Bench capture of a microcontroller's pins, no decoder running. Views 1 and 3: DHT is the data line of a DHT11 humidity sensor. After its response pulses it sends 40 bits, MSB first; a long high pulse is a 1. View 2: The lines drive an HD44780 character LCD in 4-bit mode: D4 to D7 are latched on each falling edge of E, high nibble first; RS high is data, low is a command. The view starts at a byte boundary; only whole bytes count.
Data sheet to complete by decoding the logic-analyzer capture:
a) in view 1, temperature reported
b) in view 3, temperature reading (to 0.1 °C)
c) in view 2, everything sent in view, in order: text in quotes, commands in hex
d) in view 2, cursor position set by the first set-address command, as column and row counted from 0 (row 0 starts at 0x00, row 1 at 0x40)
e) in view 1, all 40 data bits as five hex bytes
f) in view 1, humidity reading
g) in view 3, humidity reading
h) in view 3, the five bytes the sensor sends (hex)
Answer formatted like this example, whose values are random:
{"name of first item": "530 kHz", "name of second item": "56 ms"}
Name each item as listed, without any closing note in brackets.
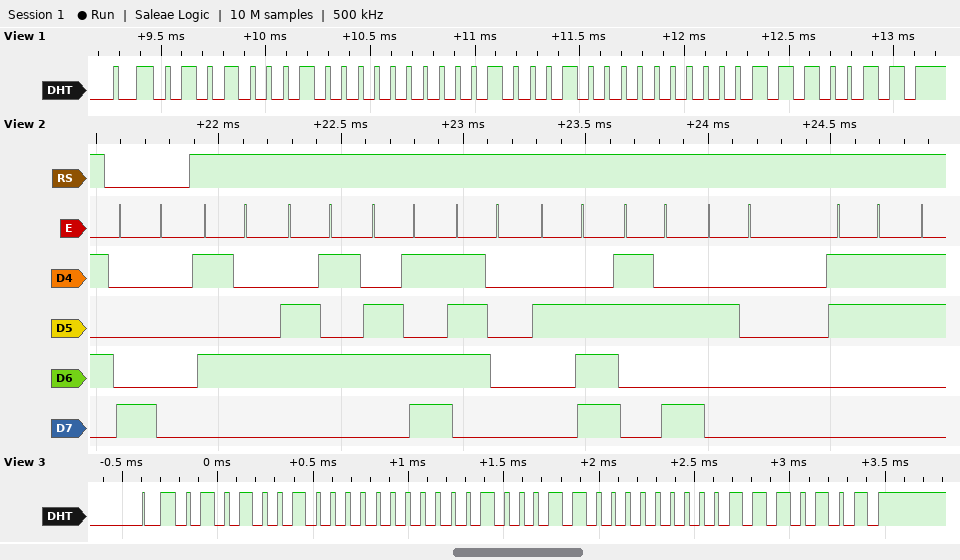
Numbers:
{"in view 1, temperature reported": "34.0 °C", "in view 3, temperature reading": "35.0 °C", "in view 2, everything sent in view, in order: text in quotes, commands in hex": "0x80 \"Temp.: 3\"", "in view 2, cursor position set by the first set-address command, as column and row counted from 0": "column 0, row 0", "in view 1, all 40 data bits as five hex bytes": "51 00 22 00 73", "in view 1, humidity reading": "81 %", "in view 3, humidity reading": "82 %", "in view 3, the five bytes the sensor sends": "52 00 23 00 75"}
